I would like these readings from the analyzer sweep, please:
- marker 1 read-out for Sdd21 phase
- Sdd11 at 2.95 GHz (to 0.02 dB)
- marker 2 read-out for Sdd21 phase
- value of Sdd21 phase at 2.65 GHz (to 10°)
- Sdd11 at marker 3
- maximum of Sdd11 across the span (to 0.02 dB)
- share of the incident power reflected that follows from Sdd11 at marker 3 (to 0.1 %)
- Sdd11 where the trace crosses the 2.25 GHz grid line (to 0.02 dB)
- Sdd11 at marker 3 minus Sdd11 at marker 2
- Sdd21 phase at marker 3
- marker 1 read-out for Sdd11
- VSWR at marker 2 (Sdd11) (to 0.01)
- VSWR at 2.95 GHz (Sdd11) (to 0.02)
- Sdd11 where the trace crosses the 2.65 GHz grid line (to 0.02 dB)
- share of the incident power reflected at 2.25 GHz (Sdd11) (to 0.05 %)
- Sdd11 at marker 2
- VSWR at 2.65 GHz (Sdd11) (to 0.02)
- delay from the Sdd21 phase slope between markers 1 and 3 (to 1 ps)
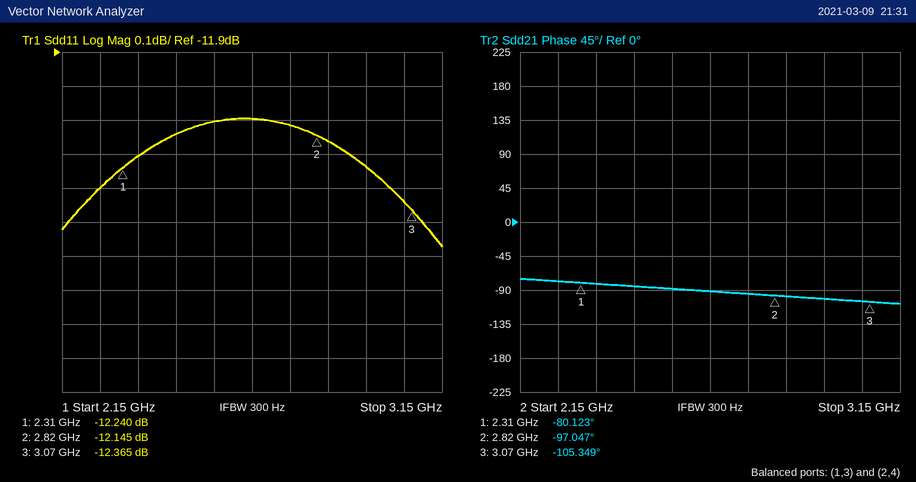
-80.123°
-12.24 dB
-97.047°
-90°
-12.365 dB
-12.10 dB
5.8 %
-12.30 dB
-0.220 dB
-105.349°
-12.240 dB
1.66
1.64
-12.10 dB
5.90 %
-12.145 dB
1.66
92 ps
